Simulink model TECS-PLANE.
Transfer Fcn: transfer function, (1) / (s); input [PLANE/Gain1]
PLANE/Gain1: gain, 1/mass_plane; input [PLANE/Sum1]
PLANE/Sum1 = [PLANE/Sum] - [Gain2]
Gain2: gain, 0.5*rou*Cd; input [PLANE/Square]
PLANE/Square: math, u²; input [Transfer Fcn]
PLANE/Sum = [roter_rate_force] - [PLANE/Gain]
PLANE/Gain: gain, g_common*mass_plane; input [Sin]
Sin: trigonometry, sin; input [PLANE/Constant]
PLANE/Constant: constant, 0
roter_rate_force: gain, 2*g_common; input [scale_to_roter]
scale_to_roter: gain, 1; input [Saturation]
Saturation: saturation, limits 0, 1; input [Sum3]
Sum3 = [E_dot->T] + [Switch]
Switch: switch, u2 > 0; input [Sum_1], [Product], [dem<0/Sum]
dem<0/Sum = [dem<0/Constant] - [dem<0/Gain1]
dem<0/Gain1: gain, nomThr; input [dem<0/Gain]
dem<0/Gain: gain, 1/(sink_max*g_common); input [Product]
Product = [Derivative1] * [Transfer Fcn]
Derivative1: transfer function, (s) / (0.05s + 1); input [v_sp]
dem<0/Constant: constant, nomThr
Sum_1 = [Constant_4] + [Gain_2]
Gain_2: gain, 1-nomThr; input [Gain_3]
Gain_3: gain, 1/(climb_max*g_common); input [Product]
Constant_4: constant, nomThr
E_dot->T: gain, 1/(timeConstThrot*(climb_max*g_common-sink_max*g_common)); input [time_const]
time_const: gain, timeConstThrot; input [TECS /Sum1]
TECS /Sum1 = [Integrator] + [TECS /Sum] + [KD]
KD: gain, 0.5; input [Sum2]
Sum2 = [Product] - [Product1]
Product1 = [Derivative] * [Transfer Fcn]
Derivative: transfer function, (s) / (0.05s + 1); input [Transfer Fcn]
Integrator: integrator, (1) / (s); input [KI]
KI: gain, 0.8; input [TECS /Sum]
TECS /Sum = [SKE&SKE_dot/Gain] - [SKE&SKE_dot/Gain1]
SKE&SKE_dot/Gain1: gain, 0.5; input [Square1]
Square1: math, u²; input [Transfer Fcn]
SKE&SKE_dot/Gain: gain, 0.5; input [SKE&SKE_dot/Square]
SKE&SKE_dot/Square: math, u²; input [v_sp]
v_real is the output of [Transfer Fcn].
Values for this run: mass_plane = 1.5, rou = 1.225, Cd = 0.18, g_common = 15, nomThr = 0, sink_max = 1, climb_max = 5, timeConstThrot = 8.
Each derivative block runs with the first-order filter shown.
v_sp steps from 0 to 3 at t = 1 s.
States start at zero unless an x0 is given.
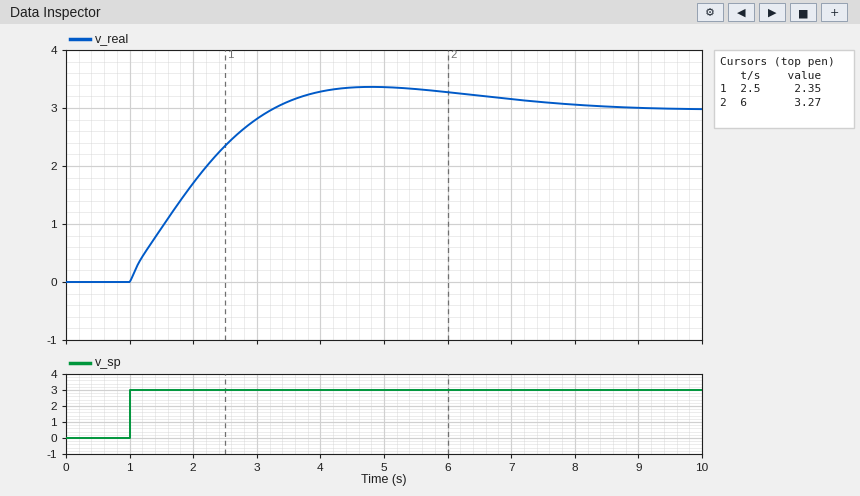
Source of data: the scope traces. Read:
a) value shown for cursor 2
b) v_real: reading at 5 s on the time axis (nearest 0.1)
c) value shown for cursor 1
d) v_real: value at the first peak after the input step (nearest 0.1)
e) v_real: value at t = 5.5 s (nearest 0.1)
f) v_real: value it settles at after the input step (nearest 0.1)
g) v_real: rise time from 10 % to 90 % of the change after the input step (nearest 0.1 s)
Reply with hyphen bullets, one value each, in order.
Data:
- 3.27
- 3.4
- 2.35
- 3.4
- 3.3
- 3.0
- 1.7 s
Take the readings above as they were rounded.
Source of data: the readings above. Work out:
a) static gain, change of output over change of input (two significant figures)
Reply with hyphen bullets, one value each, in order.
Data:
- 1.0
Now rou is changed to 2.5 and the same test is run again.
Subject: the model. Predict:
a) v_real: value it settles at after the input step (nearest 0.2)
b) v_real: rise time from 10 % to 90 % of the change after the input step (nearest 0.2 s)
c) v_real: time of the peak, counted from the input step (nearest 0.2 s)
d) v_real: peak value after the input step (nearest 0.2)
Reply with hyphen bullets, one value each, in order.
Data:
- 3.0
- 2.0 s
- 4.4 s
- 3.2
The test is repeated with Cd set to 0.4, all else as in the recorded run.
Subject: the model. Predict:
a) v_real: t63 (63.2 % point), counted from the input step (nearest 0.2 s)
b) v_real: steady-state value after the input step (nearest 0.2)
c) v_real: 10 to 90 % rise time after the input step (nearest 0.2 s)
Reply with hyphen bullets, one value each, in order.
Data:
- 1.2 s
- 3.0
- 2.0 s
